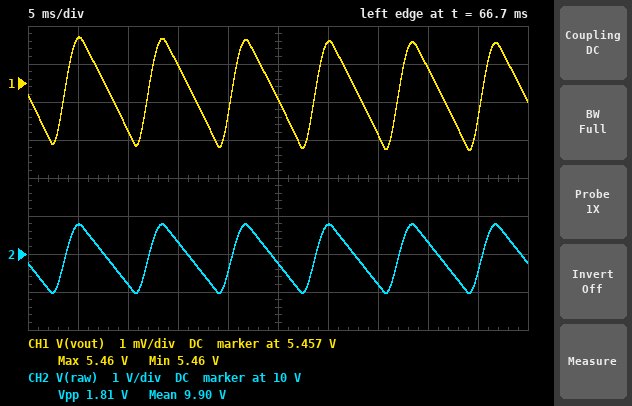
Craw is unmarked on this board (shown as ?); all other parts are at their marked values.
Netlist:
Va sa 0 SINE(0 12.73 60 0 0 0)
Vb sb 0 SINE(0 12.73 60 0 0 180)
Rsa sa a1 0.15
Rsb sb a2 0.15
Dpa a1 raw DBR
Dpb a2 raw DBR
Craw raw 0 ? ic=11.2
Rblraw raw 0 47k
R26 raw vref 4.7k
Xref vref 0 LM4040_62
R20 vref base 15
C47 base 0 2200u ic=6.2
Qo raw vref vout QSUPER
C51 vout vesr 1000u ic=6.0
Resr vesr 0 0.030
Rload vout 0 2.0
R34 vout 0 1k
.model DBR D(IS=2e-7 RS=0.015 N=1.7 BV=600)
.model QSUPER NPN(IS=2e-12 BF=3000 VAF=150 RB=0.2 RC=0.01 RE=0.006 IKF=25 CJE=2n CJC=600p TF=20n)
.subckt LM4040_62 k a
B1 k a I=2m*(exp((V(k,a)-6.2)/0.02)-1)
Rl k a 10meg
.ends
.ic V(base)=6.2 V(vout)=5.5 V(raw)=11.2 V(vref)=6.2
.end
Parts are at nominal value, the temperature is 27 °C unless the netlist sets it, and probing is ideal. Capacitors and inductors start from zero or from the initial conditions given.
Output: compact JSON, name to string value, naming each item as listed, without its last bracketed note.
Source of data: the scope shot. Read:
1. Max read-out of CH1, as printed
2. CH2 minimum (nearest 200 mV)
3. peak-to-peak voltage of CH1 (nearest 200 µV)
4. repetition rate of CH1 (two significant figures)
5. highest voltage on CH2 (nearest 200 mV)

{"Max read-out of CH1, as printed": "5.46 V", "CH2 minimum": "9.0 V", "peak-to-peak voltage of CH1": "3.0 mV", "repetition rate of CH1": "120 Hz", "highest voltage on CH2": "10.8 V"}
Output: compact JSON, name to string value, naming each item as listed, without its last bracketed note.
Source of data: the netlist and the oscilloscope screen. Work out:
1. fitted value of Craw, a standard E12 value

{"fitted value of Craw, a standard E12 value": "8.2 mF"}
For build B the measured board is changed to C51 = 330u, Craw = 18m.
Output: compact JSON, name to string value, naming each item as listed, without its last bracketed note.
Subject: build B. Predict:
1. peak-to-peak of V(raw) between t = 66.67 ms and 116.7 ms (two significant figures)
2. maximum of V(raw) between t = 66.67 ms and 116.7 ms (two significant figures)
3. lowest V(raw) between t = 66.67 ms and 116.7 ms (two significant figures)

{"peak-to-peak of V(raw) between t = 66.67 ms and 116.7 ms": "830 mV", "maximum of V(raw) between t = 66.67 ms and 116.7 ms": "10 V", "lowest V(raw) between t = 66.67 ms and 116.7 ms": "9.6 V"}
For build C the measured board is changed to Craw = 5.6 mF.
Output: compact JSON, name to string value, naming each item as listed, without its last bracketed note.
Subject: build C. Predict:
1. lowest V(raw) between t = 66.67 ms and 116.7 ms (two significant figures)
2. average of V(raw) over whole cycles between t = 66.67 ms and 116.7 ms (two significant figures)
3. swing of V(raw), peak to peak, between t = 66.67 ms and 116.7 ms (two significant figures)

{"lowest V(raw) between t = 66.67 ms and 116.7 ms": "8.4 V", "average of V(raw) over whole cycles between t = 66.67 ms and 116.7 ms": "9.7 V", "swing of V(raw), peak to peak, between t = 66.67 ms and 116.7 ms": "2.6 V"}
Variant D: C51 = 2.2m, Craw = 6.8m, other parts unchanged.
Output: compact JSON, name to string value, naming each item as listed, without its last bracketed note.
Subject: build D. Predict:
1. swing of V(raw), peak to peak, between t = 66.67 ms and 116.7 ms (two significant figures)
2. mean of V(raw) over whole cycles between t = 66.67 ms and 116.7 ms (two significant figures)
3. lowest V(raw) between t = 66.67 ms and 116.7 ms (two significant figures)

{"swing of V(raw), peak to peak, between t = 66.67 ms and 116.7 ms": "2.2 V", "mean of V(raw) over whole cycles between t = 66.67 ms and 116.7 ms": "9.8 V", "lowest V(raw) between t = 66.67 ms and 116.7 ms": "8.7 V"}
